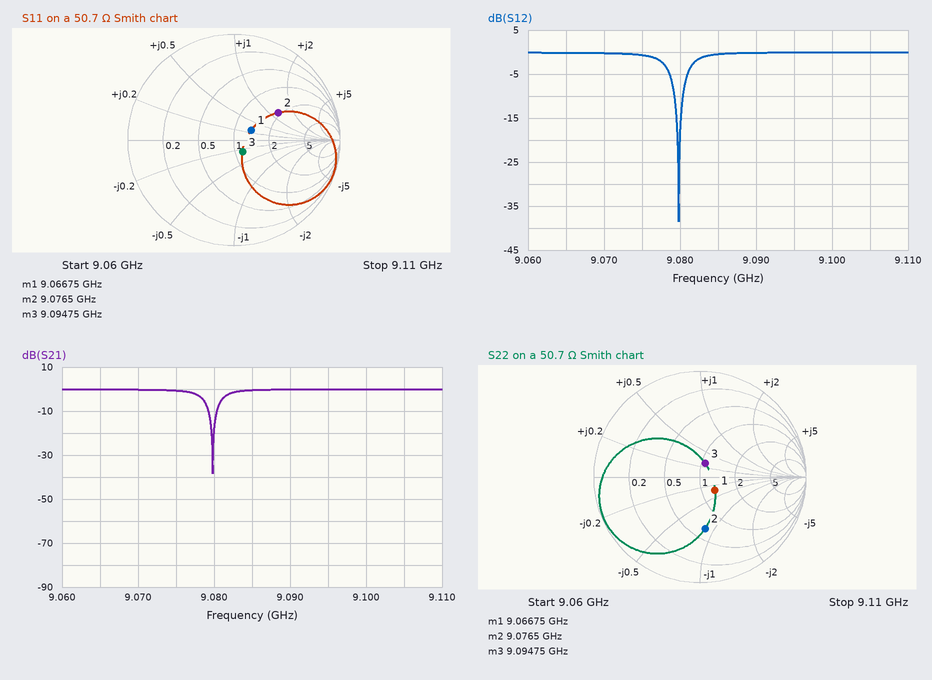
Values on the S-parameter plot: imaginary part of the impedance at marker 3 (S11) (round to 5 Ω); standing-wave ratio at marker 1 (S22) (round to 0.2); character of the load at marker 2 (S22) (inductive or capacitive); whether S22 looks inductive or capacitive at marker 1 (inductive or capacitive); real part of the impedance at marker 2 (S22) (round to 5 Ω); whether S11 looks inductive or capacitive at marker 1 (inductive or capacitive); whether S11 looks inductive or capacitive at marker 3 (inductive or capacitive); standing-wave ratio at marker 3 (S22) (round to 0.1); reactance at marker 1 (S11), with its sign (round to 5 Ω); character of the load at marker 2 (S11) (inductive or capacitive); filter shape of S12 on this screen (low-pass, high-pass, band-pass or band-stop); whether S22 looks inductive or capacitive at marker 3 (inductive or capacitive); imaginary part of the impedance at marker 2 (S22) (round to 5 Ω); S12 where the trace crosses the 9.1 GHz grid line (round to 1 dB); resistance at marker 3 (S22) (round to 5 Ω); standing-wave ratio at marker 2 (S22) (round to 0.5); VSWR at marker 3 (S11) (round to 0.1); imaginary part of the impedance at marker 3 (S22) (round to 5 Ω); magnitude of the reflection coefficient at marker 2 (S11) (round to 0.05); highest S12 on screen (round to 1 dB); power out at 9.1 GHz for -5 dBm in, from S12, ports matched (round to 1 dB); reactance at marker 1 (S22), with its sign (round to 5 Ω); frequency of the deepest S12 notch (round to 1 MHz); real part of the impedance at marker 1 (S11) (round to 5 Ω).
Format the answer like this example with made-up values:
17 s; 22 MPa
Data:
-15 Ω; 1.4; capacitive; capacitive; 35 Ω; inductive; capacitive; 1.3; +15 Ω; inductive; band-stop; inductive; -45 Ω; 0 dB; 55 Ω; 3.0; 1.3; +15 Ω; 0.50; 0 dB; -5 dBm; -15 Ω; 9.080 GHz; 70 Ω
